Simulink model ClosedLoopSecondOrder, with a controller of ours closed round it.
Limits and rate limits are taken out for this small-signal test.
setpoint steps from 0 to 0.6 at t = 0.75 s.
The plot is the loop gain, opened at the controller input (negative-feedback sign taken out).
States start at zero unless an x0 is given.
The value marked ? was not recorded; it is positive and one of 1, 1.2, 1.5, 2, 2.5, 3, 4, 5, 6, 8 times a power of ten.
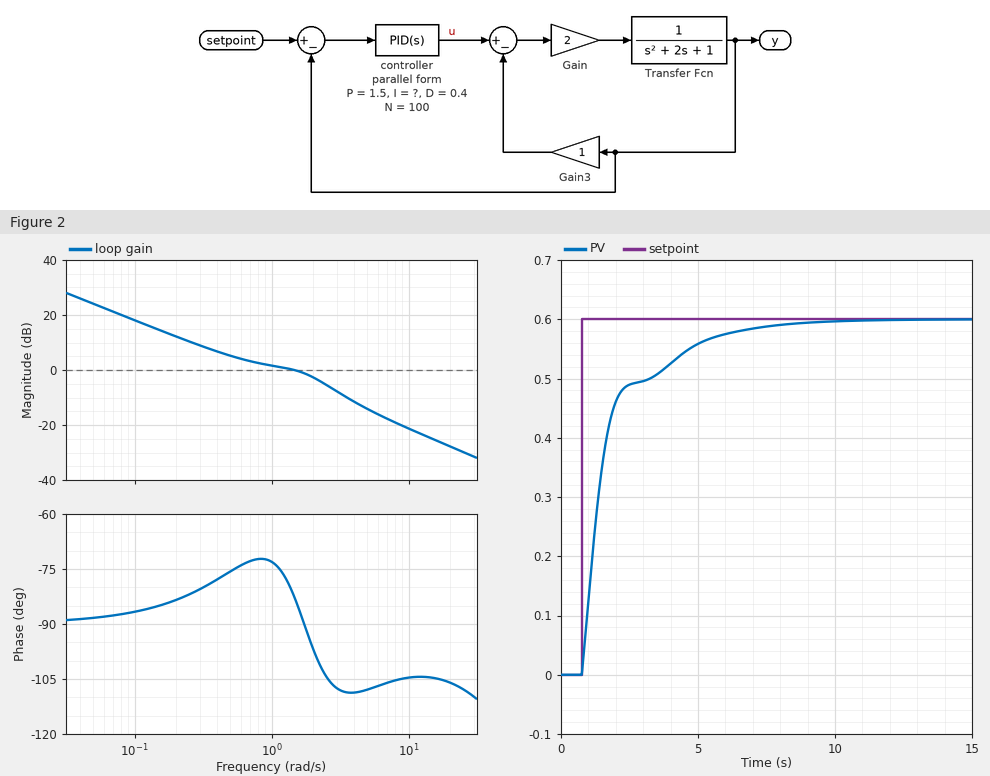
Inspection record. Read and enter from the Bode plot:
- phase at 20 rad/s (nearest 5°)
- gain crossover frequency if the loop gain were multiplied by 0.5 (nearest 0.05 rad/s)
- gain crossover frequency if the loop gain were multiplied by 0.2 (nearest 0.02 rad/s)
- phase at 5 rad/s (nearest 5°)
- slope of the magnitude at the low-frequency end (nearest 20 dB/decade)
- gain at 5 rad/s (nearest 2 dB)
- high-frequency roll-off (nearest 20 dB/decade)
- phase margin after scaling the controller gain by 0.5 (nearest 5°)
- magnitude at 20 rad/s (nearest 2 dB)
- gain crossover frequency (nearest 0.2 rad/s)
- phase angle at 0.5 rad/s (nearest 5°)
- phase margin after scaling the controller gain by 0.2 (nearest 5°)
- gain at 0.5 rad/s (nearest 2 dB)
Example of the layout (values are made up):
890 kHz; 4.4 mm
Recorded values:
-105°; 0.45 rad/s; 0.16 rad/s; -110°; -20 dB/decade; -14 dB; -20 dB/decade; 105°; -28 dB; 1.4 rad/s; -75°; 95°; 6 dB
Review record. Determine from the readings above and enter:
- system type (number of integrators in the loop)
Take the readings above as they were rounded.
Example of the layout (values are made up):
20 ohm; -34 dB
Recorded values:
1
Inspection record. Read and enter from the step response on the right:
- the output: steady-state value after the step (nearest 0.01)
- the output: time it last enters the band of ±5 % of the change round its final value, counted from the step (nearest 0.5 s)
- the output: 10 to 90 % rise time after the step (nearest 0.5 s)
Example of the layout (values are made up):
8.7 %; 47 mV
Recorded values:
0.60; 5.0 s; 3.5 s
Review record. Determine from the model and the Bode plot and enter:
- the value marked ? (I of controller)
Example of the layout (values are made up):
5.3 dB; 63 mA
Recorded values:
1.2
